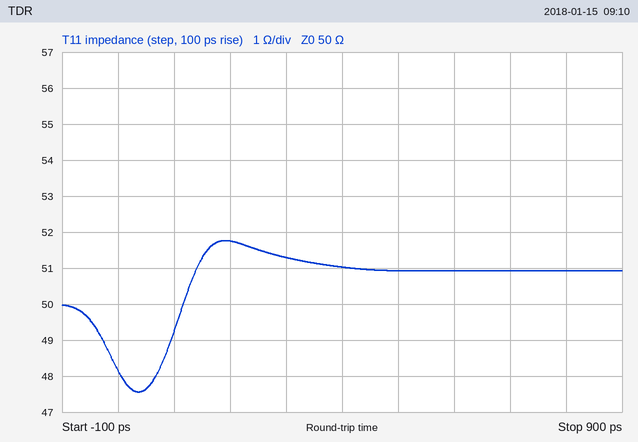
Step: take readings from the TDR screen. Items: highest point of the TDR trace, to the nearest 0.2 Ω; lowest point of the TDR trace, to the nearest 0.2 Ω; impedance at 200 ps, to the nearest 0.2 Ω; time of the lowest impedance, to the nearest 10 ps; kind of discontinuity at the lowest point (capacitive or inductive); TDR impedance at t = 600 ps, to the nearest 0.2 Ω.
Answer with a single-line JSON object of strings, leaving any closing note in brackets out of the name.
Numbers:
{"highest point of the TDR trace, to the nearest 0.2 Ω": "51.8 Ω", "lowest point of the TDR trace, to the nearest 0.2 Ω": "47.6 Ω", "impedance at 200 ps, to the nearest 0.2 Ω": "51.8 Ω", "time of the lowest impedance, to the nearest 10 ps": "40 ps", "kind of discontinuity at the lowest point": "capacitive", "TDR impedance at t = 600 ps, to the nearest 0.2 Ω": "51.0 Ω"}
